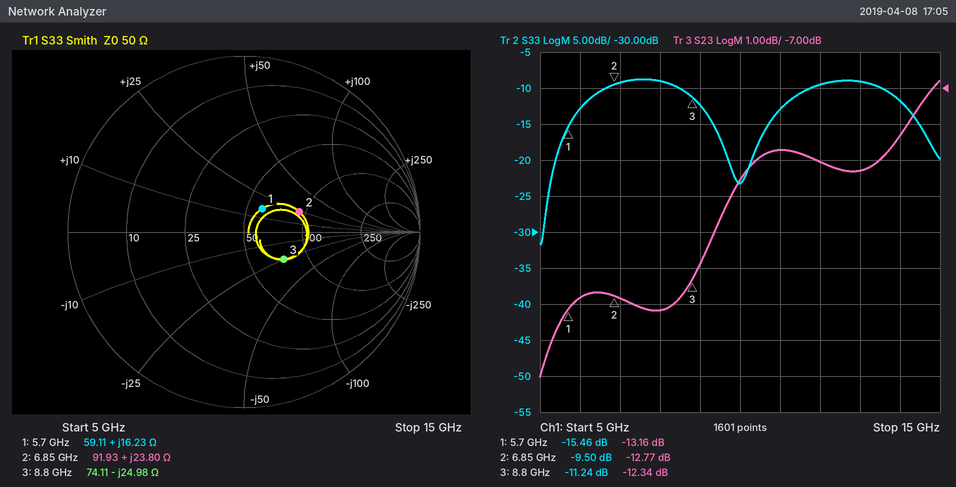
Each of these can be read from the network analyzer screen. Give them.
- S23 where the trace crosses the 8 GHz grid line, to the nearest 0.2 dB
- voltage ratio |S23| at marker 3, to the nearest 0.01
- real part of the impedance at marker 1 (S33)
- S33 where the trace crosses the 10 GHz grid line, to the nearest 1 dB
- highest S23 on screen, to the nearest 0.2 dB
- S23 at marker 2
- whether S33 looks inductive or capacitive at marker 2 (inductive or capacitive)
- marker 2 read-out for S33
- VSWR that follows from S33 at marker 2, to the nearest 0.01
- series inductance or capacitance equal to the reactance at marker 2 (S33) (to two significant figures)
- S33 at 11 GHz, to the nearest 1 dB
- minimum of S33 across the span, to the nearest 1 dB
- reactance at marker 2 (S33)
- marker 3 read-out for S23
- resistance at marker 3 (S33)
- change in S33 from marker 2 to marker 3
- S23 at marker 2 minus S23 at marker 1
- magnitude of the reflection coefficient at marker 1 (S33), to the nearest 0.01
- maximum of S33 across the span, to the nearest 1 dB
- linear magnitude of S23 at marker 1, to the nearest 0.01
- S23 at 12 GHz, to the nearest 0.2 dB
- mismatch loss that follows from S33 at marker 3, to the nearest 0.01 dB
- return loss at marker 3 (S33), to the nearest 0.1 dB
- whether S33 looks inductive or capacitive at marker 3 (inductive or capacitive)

-13.2 dB
0.24
59.11 Ω
-23 dB
-6.8 dB
-12.77 dB
inductive
-9.50 dB
2.01
550 pH
-13 dB
-32 dB
+23.80 Ω
-12.34 dB
74.11 Ω
-1.74 dB
0.39 dB
0.17
-9 dB
0.22
-9.0 dB
0.34 dB
11.2 dB
capacitive
